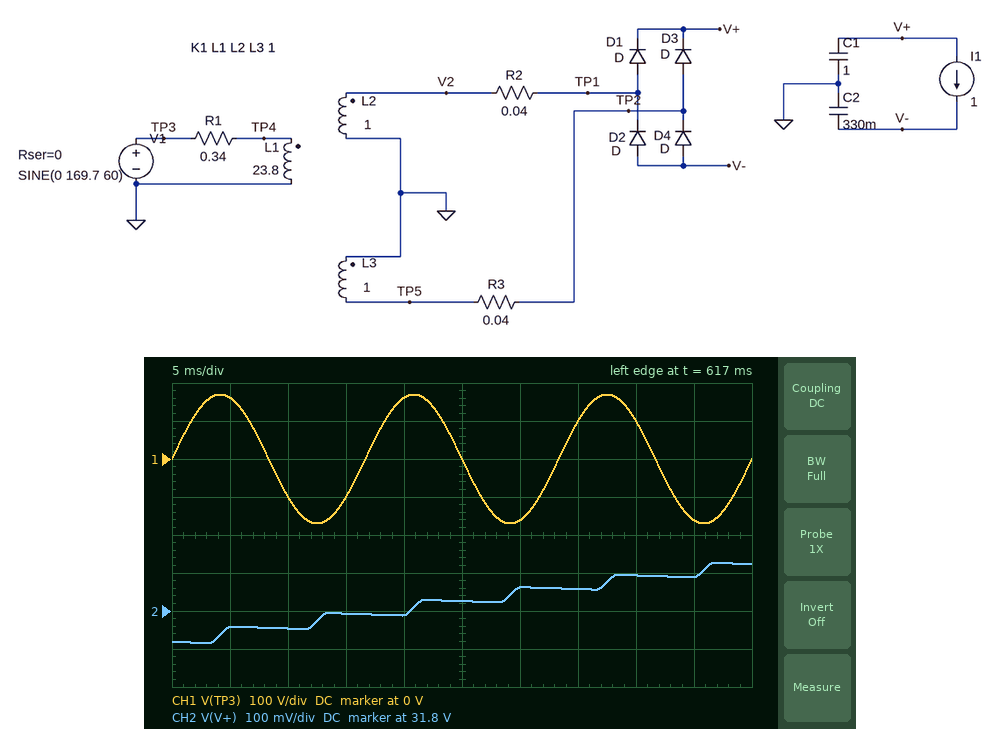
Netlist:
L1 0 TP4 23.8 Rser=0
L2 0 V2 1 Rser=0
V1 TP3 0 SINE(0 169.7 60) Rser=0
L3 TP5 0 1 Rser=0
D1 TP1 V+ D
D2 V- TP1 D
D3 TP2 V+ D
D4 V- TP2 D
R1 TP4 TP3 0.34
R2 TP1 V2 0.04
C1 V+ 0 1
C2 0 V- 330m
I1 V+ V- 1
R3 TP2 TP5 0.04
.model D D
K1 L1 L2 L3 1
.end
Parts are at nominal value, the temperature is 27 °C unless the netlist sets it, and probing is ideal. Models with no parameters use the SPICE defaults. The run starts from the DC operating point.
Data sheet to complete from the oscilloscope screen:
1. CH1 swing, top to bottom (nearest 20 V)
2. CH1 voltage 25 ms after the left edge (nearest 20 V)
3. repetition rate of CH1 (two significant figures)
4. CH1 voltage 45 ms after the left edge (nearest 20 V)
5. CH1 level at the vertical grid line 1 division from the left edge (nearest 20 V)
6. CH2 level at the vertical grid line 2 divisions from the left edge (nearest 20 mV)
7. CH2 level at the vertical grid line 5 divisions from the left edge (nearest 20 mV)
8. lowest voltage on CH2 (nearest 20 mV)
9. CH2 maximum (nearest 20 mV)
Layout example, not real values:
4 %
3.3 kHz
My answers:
340 V
0 V
60 Hz
-160 V
160 V
31.76 V
31.82 V
31.72 V
31.92 V
